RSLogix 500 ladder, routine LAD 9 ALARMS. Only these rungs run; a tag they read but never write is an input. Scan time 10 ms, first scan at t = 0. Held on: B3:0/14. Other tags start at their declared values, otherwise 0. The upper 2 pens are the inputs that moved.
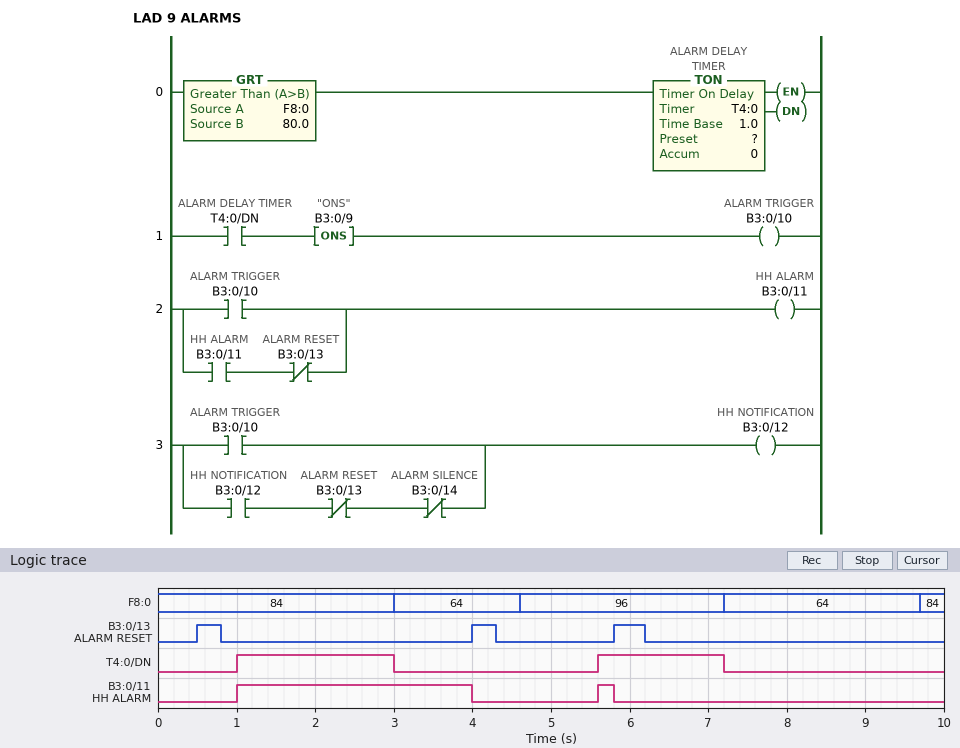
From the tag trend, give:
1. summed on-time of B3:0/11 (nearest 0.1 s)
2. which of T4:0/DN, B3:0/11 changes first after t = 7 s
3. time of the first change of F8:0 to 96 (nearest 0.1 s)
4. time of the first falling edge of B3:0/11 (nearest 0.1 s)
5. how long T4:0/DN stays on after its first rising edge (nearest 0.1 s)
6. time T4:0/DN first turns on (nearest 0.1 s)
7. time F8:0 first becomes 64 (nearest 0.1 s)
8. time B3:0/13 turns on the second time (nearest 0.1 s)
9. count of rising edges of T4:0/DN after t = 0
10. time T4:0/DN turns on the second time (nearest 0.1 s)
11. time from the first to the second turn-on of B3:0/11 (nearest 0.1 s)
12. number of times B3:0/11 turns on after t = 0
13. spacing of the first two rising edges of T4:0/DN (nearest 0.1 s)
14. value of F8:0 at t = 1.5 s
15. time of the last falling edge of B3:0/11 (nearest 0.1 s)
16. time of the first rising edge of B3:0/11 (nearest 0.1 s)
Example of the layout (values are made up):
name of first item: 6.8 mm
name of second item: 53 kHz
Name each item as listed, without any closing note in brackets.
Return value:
summed on-time of B3:0/11: 3.2 s
which of T4:0/DN, B3:0/11 changes first after t = 7 s: T4:0/DN
time of the first change of F8:0 to 96: 4.6 s
time of the first falling edge of B3:0/11: 4.0 s
how long T4:0/DN stays on after its first rising edge: 2.0 s
time T4:0/DN first turns on: 1.0 s
time F8:0 first becomes 64: 3.0 s
time B3:0/13 turns on the second time: 4.0 s
count of rising edges of T4:0/DN after t = 0: 2
time T4:0/DN turns on the second time: 5.6 s
time from the first to the second turn-on of B3:0/11: 4.6 s
number of times B3:0/11 turns on after t = 0: 2
spacing of the first two rising edges of T4:0/DN: 4.6 s
value of F8:0 at t = 1.5 s: 84
time of the last falling edge of B3:0/11: 5.8 s
time of the first rising edge of B3:0/11: 1.0 s
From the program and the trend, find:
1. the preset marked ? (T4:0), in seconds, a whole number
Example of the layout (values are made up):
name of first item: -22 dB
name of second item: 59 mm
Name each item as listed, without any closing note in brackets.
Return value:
the preset marked ? (T4:0), in seconds, a whole number: 1 s
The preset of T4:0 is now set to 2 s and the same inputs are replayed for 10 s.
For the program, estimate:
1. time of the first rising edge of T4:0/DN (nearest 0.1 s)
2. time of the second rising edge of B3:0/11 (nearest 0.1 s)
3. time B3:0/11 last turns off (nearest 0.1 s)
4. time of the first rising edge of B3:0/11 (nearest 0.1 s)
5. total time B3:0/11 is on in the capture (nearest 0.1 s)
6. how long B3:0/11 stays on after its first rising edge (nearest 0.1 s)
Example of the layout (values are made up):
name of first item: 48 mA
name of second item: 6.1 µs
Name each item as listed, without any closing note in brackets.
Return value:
time of the first rising edge of T4:0/DN: 2.0 s
time of the second rising edge of B3:0/11: 6.6 s
time B3:0/11 last turns off: 4.0 s
time of the first rising edge of B3:0/11: 2.0 s
total time B3:0/11 is on in the capture: 5.4 s
how long B3:0/11 stays on after its first rising edge: 2.0 s
